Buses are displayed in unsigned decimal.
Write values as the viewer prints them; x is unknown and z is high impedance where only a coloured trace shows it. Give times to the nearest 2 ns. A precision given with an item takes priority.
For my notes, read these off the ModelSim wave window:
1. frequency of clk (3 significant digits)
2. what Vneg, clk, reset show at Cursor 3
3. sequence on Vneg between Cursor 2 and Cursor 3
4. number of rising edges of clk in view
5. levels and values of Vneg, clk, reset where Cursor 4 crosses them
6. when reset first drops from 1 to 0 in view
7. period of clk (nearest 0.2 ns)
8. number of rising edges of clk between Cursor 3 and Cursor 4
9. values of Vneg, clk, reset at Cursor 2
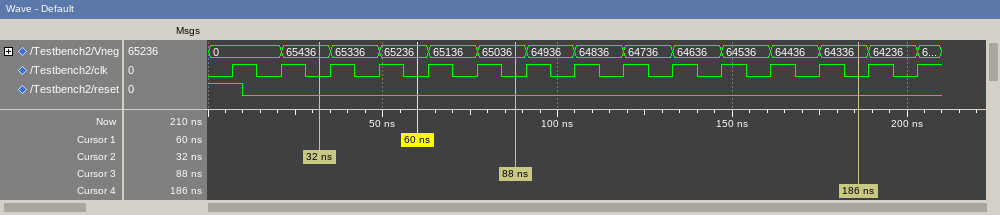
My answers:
71.4 MHz
Vneg=65036, clk=0, reset=0
65436, 65336, 65236, 65136, 65036
15
Vneg=64336, clk=0, reset=0
10 ns
14 ns
7
Vneg=65436, clk=0, reset=0
